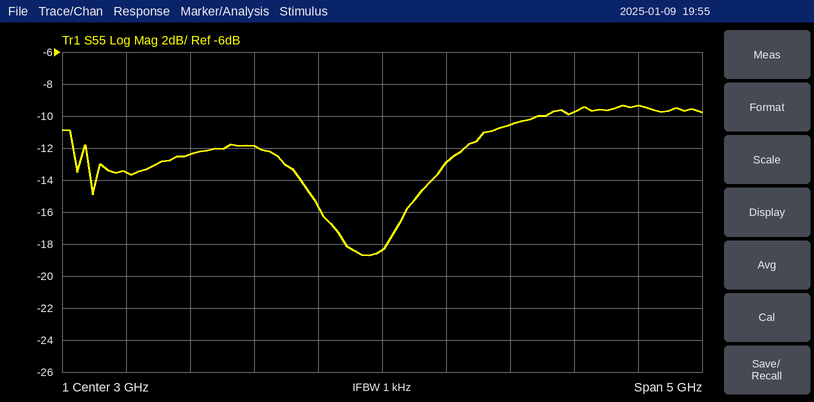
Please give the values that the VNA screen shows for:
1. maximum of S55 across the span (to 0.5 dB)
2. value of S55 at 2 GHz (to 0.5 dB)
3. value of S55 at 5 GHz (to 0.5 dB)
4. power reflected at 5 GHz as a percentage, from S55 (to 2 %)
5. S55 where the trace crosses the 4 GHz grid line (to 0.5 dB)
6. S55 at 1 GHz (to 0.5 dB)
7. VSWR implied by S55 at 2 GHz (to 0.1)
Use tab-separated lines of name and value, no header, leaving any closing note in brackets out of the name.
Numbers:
maximum of S55 across the span	-9.5 dB
value of S55 at 2 GHz	-12.0 dB
value of S55 at 5 GHz	-9.5 dB
power reflected at 5 GHz as a percentage, from S55	12 %
S55 where the trace crosses the 4 GHz grid line	-10.5 dB
S55 at 1 GHz	-13.5 dB
VSWR implied by S55 at 2 GHz	1.7
